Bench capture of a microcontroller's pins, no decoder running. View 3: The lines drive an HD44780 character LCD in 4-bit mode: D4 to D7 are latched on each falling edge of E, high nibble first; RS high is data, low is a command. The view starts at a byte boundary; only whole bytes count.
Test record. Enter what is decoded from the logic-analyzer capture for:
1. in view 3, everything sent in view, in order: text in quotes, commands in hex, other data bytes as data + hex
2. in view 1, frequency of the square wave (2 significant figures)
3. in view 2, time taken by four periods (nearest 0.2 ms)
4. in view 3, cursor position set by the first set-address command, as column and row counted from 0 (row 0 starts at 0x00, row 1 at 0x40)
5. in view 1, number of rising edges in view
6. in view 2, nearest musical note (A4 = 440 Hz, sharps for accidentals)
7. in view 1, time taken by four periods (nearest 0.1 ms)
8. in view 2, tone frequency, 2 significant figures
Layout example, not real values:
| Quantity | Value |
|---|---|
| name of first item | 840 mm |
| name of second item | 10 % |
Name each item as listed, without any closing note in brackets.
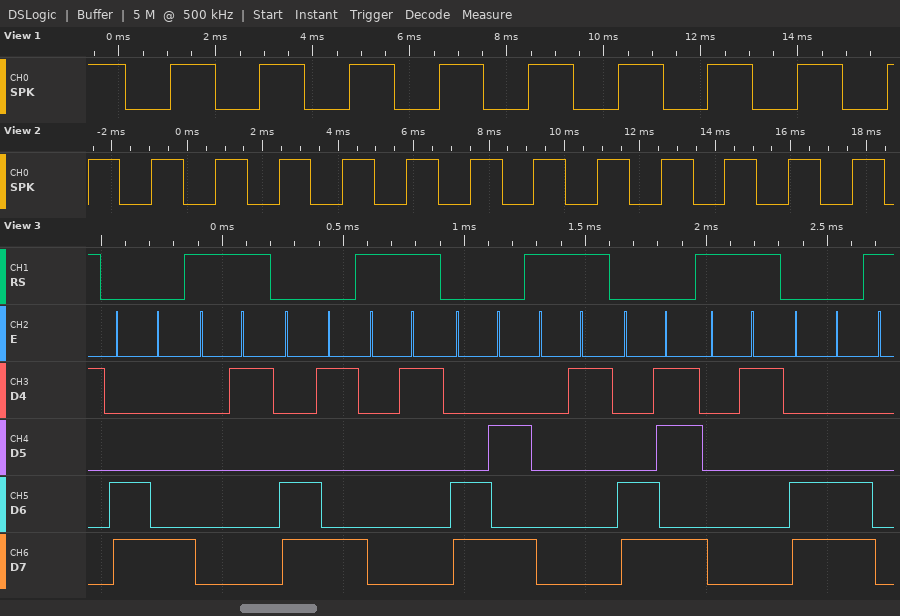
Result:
| Quantity | Value |
|---|---|
| in view 3, everything sent in view, in order: text in quotes, commands in hex, other data bytes as data + hex | 0xC8 data 01 0xC9 data 01 0xCA data 01 0xCB data 01 0xCC |
| in view 1, frequency of the square wave | 540 Hz |
| in view 2, time taken by four periods | 6.8 ms |
| in view 3, cursor position set by the first set-address command, as column and row counted from 0 | column 8, row 1 |
| in view 1, number of rising edges in view | 9 |
| in view 2, nearest musical note | D5 |
| in view 1, time taken by four periods | 7.4 ms |
| in view 2, tone frequency, 2 significant figures | 590 Hz |
